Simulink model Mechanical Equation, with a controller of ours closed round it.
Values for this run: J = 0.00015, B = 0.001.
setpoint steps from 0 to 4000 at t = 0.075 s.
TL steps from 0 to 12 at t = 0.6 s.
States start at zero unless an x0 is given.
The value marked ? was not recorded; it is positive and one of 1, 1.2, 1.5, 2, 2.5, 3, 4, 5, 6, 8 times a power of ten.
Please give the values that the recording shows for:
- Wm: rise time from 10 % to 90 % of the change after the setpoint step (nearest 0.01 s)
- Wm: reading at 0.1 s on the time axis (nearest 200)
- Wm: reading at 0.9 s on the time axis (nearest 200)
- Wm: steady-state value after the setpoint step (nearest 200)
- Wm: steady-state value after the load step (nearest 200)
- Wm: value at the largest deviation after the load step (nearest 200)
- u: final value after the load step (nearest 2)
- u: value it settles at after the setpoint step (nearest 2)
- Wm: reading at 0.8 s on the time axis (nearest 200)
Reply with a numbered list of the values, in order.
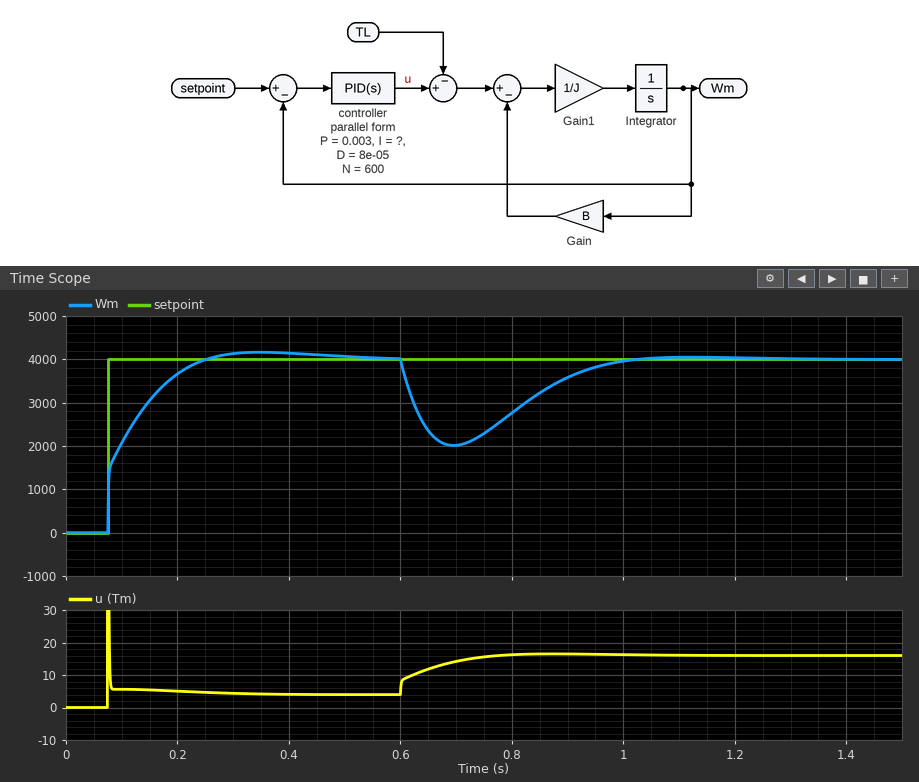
1. 0.12 s
2. 2000
3. 3600
4. 4000
5. 4000
6. 2000
7. 16
8. 4
9. 2800
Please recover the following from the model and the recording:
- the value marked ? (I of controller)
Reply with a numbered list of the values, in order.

1. 0.03
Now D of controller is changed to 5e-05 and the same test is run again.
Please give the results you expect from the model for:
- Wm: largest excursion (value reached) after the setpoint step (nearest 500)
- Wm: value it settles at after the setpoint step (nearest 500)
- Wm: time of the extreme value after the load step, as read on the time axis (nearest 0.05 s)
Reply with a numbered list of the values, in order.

1. 4000
2. 4000
3. 0.70 s
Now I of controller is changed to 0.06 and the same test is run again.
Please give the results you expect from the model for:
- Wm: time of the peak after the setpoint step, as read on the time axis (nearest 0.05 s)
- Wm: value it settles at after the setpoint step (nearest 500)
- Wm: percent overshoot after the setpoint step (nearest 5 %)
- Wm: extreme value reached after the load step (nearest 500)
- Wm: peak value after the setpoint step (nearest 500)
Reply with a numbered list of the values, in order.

1. 0.25 s
2. 4000
3. 10 %
4. 2500
5. 4500
